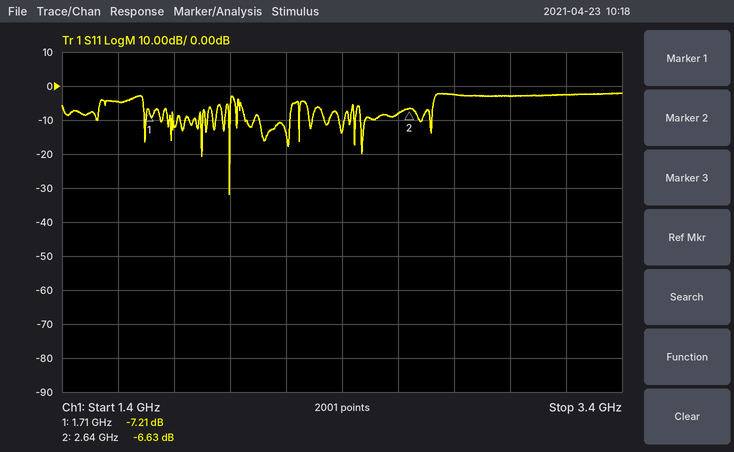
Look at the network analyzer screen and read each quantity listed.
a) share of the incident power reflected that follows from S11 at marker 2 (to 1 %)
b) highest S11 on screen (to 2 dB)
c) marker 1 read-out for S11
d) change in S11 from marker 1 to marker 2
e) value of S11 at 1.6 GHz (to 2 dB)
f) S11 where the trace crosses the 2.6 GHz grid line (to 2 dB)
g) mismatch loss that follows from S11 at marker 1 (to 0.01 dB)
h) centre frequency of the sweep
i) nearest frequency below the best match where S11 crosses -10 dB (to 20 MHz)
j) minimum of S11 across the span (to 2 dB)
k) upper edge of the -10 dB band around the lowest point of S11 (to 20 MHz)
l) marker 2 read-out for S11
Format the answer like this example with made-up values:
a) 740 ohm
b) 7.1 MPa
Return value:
a) 22 %
b) -2 dB
c) -7.21 dB
d) 0.58 dB
e) -4 dB
f) -8 dB
g) 0.92 dB
h) 2.4 GHz
i) 2.00 GHz
j) -32 dB
k) 2.00 GHz
l) -6.63 dB
